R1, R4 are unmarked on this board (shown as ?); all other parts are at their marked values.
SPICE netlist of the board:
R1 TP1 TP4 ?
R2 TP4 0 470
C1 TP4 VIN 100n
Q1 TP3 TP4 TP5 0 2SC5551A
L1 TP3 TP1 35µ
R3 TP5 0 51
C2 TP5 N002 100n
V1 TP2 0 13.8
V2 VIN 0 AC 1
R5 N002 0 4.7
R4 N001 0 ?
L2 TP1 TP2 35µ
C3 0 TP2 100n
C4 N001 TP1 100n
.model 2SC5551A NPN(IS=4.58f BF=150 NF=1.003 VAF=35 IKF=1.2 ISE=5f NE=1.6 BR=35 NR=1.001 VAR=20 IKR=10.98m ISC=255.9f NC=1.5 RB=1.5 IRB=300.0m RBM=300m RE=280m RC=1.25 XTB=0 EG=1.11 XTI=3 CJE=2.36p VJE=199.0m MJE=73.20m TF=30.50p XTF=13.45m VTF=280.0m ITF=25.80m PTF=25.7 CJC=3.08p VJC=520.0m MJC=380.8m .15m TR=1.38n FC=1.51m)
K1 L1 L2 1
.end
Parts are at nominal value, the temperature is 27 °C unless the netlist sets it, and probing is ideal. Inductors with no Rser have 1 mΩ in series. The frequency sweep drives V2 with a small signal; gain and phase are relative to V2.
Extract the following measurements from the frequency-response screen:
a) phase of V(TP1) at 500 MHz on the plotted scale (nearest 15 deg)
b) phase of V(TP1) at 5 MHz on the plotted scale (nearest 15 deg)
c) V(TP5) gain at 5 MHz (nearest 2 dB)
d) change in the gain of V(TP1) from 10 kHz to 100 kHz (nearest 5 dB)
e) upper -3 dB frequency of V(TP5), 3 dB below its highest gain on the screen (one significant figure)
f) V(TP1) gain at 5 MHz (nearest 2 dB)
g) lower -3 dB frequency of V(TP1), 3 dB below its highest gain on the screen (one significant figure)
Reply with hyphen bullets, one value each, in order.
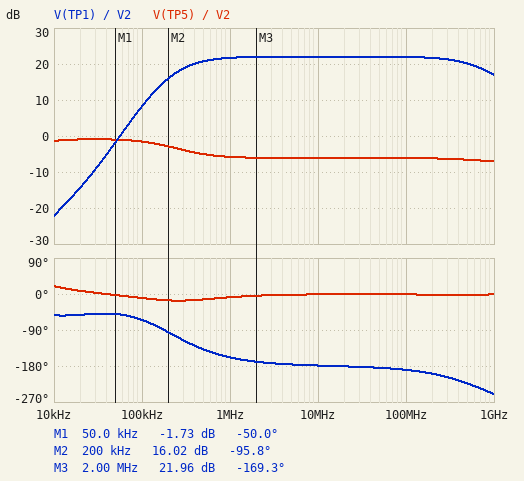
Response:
- -225 deg
- -180 deg
- -6 dB
- 30 dB
- 300 kHz
- 22 dB
- 300 kHz
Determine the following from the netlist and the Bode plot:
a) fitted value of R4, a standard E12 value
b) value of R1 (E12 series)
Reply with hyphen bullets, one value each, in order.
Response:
- 56 Ω
- 5.6 kΩ
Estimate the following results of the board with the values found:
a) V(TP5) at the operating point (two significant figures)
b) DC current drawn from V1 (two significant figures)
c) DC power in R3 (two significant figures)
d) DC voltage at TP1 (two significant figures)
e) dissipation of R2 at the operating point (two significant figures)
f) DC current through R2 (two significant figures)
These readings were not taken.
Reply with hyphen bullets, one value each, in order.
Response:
- 330 mV
- 8.8 mA
- 2.2 mW
- 14 V
- 2.4 mW
- 2.2 mA
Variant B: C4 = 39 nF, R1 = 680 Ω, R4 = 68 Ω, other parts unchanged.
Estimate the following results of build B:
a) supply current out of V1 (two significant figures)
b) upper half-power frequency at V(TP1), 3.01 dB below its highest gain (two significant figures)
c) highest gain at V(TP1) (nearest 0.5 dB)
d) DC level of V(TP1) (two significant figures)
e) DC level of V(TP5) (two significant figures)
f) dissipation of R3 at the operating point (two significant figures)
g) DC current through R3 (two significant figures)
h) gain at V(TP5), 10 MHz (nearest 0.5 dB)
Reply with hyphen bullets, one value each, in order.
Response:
- 100 mA
- 470 MHz
- 27.5 dB
- 14 V
- 4.7 V
- 430 mW
- 92 mA
- -1.5 dB
